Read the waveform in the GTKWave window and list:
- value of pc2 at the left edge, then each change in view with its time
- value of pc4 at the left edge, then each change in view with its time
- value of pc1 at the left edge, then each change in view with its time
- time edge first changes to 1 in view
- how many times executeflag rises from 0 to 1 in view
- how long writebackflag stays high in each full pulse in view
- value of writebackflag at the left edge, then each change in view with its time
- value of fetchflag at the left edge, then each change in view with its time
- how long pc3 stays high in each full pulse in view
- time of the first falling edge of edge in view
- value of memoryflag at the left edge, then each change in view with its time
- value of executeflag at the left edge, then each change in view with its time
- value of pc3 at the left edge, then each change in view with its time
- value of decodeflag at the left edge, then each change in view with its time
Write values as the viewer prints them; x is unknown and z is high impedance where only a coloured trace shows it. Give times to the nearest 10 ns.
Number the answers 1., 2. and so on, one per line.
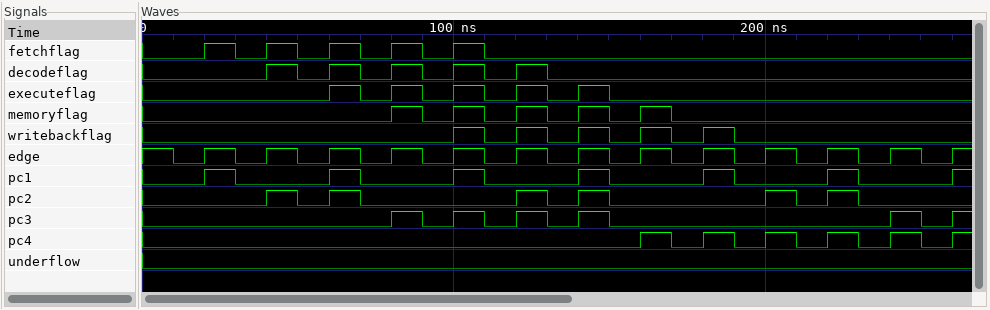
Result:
1. 0, 1 at 40 ns, 0 at 50 ns, 1 at 60 ns, 0 at 70 ns, 1 at 120 ns, 0 at 130 ns, 1 at 140 ns, 0 at 150 ns, 1 at 200 ns, 0 at 210 ns, 1 at 220 ns, 0 at 230 ns
2. 0, 1 at 160 ns, 0 at 170 ns, 1 at 180 ns, 0 at 190 ns, 1 at 200 ns, 0 at 210 ns, 1 at 220 ns, 0 at 230 ns, 1 at 240 ns, 0 at 250 ns, 1 at 260 ns
3. 0, 1 at 20 ns, 0 at 30 ns, 1 at 60 ns, 0 at 70 ns, 1 at 100 ns, 0 at 110 ns, 1 at 140 ns, 0 at 150 ns, 1 at 180 ns, 0 at 190 ns, 1 at 220 ns, 0 at 230 ns, 1 at 260 ns
4. 20 ns
5. 5
6. 10 ns, 10 ns, 10 ns, 10 ns, 10 ns
7. 0, 1 at 100 ns, 0 at 110 ns, 1 at 120 ns, 0 at 130 ns, 1 at 140 ns, 0 at 150 ns, 1 at 160 ns, 0 at 170 ns, 1 at 180 ns, 0 at 190 ns
8. 0, 1 at 20 ns, 0 at 30 ns, 1 at 40 ns, 0 at 50 ns, 1 at 60 ns, 0 at 70 ns, 1 at 80 ns, 0 at 90 ns, 1 at 100 ns, 0 at 110 ns
9. 10 ns, 10 ns, 10 ns, 10 ns, 10 ns
10. 10 ns
11. 0, 1 at 80 ns, 0 at 90 ns, 1 at 100 ns, 0 at 110 ns, 1 at 120 ns, 0 at 130 ns, 1 at 140 ns, 0 at 150 ns, 1 at 160 ns, 0 at 170 ns
12. 0, 1 at 60 ns, 0 at 70 ns, 1 at 80 ns, 0 at 90 ns, 1 at 100 ns, 0 at 110 ns, 1 at 120 ns, 0 at 130 ns, 1 at 140 ns, 0 at 150 ns
13. 0, 1 at 80 ns, 0 at 90 ns, 1 at 100 ns, 0 at 110 ns, 1 at 120 ns, 0 at 130 ns, 1 at 140 ns, 0 at 150 ns, 1 at 240 ns, 0 at 250 ns, 1 at 260 ns
14. 0, 1 at 40 ns, 0 at 50 ns, 1 at 60 ns, 0 at 70 ns, 1 at 80 ns, 0 at 90 ns, 1 at 100 ns, 0 at 110 ns, 1 at 120 ns, 0 at 130 ns
